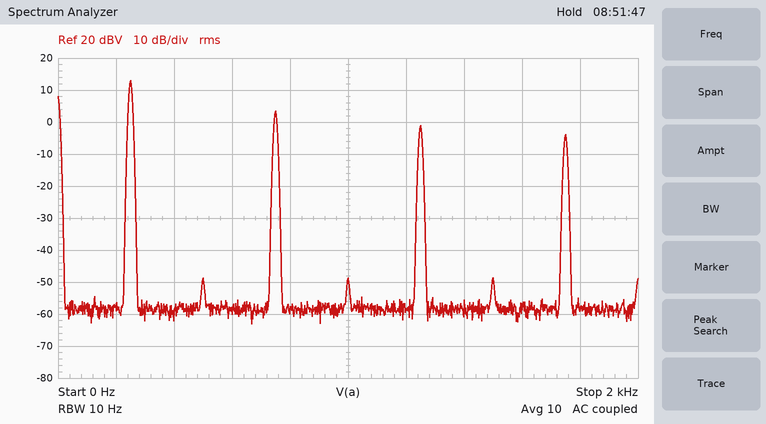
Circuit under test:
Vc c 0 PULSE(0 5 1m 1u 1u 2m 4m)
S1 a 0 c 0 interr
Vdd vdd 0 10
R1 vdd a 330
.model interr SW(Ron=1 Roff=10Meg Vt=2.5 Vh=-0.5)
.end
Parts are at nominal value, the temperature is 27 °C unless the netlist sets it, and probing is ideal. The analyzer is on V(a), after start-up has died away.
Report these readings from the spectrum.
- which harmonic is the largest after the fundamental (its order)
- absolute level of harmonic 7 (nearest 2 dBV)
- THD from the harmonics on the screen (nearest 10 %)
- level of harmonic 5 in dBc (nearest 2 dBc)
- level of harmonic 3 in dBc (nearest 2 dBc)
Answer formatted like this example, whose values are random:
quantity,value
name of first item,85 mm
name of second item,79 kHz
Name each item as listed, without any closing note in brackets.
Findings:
quantity,value
which harmonic is the largest after the fundamental,3
absolute level of harmonic 7,-4 dBV
THD from the harmonics on the screen,40 %
level of harmonic 5 in dBc,-14 dBc
level of harmonic 3 in dBc,-10 dBc
